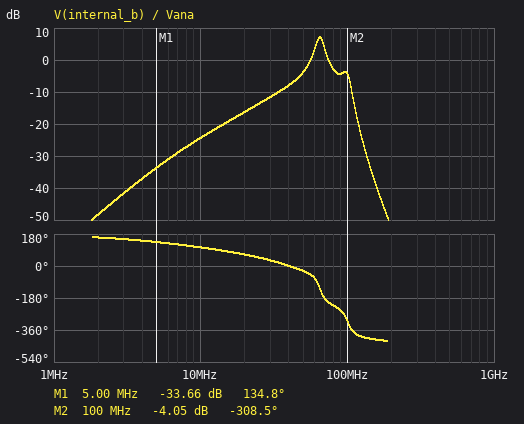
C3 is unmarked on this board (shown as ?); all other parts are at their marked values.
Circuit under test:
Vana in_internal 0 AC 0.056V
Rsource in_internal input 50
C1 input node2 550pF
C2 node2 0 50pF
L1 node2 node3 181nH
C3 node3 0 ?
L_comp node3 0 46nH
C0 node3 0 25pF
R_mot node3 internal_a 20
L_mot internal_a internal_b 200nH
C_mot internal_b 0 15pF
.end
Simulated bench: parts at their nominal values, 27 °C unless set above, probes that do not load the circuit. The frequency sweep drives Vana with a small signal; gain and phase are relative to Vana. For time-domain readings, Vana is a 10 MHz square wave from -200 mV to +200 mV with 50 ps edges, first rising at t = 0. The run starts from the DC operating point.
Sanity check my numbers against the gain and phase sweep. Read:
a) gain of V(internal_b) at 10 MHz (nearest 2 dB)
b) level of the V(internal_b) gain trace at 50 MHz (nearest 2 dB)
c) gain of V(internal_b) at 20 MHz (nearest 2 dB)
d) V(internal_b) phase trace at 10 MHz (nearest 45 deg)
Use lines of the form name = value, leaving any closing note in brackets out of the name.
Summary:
gain of V(internal_b) at 10 MHz = -24 dB
level of the V(internal_b) gain trace at 50 MHz = -4 dB
gain of V(internal_b) at 20 MHz = -16 dB
V(internal_b) phase trace at 10 MHz = 90 deg
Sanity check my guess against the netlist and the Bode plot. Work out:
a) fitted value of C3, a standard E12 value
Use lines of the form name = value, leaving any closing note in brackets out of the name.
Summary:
fitted value of C3, a standard E12 value = 120 pF
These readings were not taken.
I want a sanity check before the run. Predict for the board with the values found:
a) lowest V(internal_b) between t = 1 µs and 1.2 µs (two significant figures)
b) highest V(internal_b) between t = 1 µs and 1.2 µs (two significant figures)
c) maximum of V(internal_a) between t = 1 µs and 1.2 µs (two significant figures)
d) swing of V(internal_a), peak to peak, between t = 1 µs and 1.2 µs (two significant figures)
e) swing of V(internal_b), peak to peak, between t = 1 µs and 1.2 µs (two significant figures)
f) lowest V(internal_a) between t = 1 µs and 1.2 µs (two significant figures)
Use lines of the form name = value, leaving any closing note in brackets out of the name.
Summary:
lowest V(internal_b) between t = 1 µs and 1.2 µs = -110 mV
highest V(internal_b) between t = 1 µs and 1.2 µs = 110 mV
maximum of V(internal_a) between t = 1 µs and 1.2 µs = 60 mV
swing of V(internal_a), peak to peak, between t = 1 µs and 1.2 µs = 120 mV
swing of V(internal_b), peak to peak, between t = 1 µs and 1.2 µs = 220 mV
lowest V(internal_a) between t = 1 µs and 1.2 µs = -60 mV
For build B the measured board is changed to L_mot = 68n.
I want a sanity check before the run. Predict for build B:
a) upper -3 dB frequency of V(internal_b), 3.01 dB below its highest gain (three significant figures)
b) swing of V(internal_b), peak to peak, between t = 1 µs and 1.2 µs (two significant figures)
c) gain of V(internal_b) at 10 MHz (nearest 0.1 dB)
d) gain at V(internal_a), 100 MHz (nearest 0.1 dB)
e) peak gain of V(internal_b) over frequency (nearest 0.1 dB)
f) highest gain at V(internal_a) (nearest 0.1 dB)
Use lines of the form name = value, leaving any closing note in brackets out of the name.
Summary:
upper -3 dB frequency of V(internal_b), 3.01 dB below its highest gain = 70.8 MHz
swing of V(internal_b), peak to peak, between t = 1 µs and 1.2 µs = 190 mV
gain of V(internal_b) at 10 MHz = -24.4 dB
gain at V(internal_a), 100 MHz = -21.0 dB
peak gain of V(internal_b) over frequency = 4.8 dB
highest gain at V(internal_a) = 3.1 dB
